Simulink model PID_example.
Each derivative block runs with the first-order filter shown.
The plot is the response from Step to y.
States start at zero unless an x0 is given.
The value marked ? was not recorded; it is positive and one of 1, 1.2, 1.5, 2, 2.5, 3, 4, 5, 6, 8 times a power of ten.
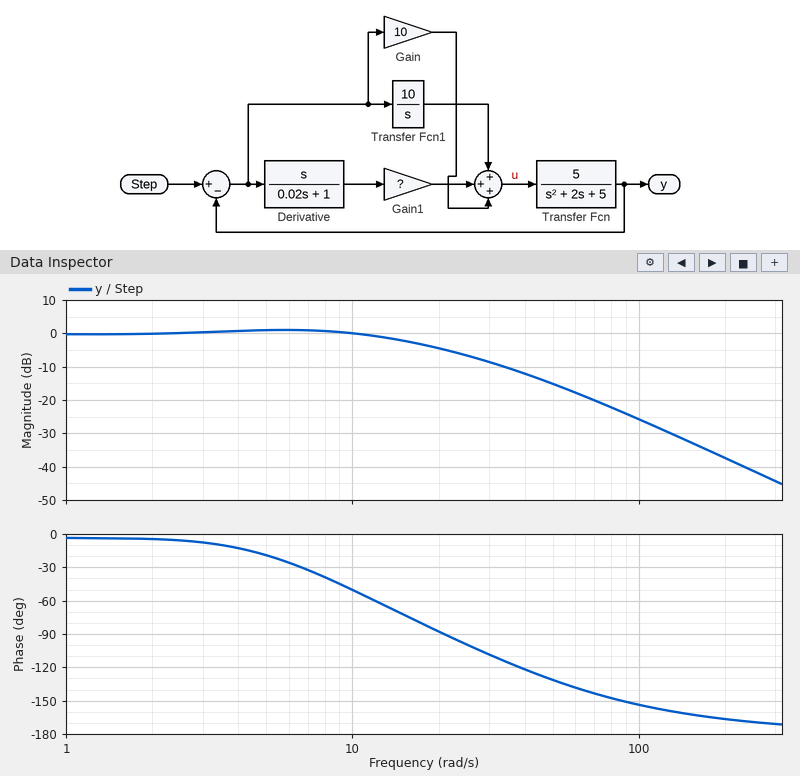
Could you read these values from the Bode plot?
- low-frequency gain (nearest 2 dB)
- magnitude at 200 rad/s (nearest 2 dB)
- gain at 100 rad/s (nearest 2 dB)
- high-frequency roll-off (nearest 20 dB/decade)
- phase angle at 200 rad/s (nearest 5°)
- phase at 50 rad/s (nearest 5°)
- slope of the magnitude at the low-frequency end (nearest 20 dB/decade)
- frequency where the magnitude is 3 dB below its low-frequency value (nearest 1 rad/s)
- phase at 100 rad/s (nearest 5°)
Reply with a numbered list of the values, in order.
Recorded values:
1. 0 dB
2. -38 dB
3. -26 dB
4. -40 dB/decade
5. -165°
6. -130°
7. 0 dB/decade
8. 17 rad/s
9. -155°
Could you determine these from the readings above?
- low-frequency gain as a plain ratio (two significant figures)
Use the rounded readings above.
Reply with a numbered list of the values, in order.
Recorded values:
1. 1.0
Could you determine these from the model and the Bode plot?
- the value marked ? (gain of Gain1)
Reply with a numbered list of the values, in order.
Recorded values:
1. 2
